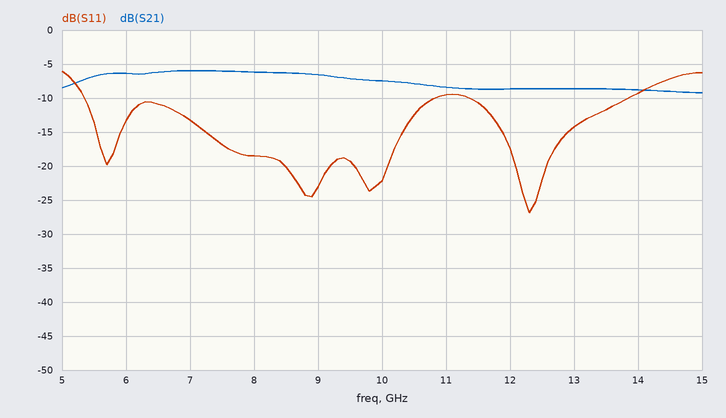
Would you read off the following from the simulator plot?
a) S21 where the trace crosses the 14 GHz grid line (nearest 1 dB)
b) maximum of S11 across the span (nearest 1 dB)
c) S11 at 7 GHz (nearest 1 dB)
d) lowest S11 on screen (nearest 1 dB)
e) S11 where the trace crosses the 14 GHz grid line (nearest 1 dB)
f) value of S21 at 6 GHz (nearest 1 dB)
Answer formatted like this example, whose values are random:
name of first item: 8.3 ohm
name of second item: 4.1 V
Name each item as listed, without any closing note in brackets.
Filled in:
S21 where the trace crosses the 14 GHz grid line: -9 dB
maximum of S11 across the span: -6 dB
S11 at 7 GHz: -13 dB
lowest S11 on screen: -27 dB
S11 where the trace crosses the 14 GHz grid line: -9 dB
value of S21 at 6 GHz: -6 dB
